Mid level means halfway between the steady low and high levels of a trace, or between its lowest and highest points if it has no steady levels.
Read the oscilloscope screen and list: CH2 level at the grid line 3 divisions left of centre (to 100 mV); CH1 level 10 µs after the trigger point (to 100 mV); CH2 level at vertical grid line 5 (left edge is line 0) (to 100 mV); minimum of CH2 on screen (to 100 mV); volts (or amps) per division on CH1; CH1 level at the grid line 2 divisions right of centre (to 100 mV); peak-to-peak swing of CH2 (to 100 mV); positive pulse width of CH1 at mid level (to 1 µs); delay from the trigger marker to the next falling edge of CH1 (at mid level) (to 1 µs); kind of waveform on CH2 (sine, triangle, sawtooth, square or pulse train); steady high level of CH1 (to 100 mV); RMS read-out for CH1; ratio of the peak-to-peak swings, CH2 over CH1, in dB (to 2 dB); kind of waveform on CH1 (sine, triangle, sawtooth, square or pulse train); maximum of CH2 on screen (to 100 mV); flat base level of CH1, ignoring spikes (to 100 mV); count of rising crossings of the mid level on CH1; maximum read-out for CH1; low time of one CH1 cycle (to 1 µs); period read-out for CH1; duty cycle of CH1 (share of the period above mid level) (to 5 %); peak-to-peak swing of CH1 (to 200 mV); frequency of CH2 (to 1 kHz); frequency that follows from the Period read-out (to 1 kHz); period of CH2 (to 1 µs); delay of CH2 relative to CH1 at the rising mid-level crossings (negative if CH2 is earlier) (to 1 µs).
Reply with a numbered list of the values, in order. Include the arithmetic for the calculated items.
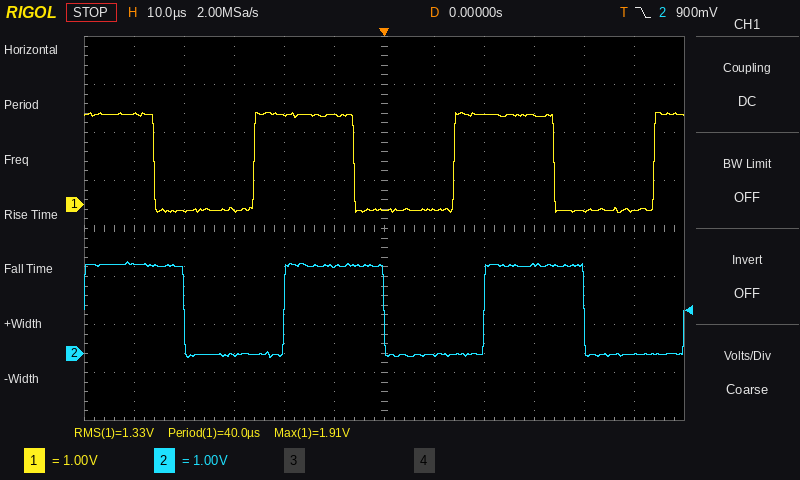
1. 0.0 V
2. -100 mV
3. 1.8 V
4. -100 mV
5. 1 V
6. 1.9 V
7. 1.9 V − (-100 mV) = 2.0 V
8. 20 µs
9. 34 µs
10. square
11. 1.9 V
12. 1.33 V
13. 20 log10(2.0 V / 2.0 V) ≈ 0 dB
14. square
15. 1.9 V
16. -100 mV
17. 3
18. 1.91 V
19. 20 µs
20. 40.0 µs
21. 50 %
22. 2.0 V
23. 1 / 40 µs ≈ 25 kHz
24. 1 / 40.0 µs ≈ 25 kHz
25. 40 µs
26. +6 µs
